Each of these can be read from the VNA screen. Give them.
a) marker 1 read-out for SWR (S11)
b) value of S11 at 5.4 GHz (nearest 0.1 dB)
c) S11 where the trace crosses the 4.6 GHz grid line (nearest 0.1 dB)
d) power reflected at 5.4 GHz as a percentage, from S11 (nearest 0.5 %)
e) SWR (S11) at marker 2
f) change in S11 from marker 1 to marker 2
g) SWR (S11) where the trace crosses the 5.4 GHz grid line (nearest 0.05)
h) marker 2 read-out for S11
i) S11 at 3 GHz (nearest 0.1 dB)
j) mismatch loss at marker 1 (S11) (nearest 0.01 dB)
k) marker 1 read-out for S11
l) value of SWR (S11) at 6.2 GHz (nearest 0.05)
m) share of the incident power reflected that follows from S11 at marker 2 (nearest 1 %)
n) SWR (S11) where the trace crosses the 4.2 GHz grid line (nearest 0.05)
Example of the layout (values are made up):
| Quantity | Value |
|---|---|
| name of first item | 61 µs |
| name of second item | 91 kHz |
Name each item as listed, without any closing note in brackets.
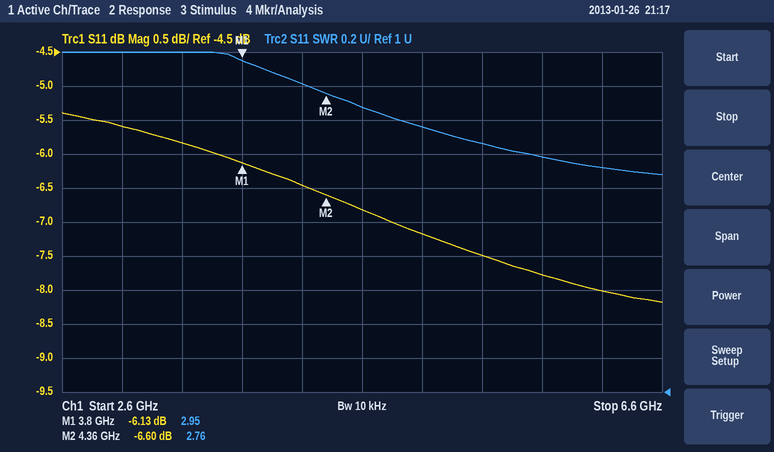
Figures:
| Quantity | Value |
|---|---|
| marker 1 read-out for SWR | 2.95 |
| value of S11 at 5.4 GHz | -7.5 dB |
| S11 where the trace crosses the 4.6 GHz grid line | -6.8 dB |
| power reflected at 5.4 GHz as a percentage, from S11 | 18.0 % |
| SWR (S11) at marker 2 | 2.76 |
| change in S11 from marker 1 to marker 2 | -0.47 dB |
| SWR (S11) where the trace crosses the 5.4 GHz grid line | 2.45 |
| marker 2 read-out for S11 | -6.60 dB |
| S11 at 3 GHz | -5.6 dB |
| mismatch loss at marker 1 (S11) | 1.21 dB |
| marker 1 read-out for S11 | -6.13 dB |
| value of SWR (S11) at 6.2 GHz | 2.30 |
| share of the incident power reflected that follows from S11 at marker 2 | 22 % |
| SWR (S11) where the trace crosses the 4.2 GHz grid line | 2.80 |
